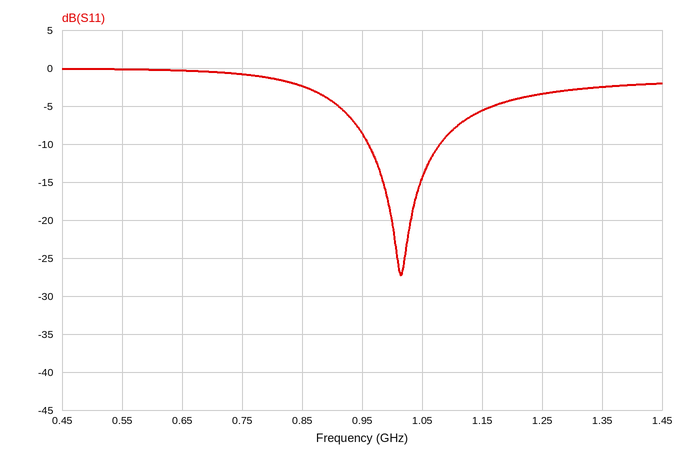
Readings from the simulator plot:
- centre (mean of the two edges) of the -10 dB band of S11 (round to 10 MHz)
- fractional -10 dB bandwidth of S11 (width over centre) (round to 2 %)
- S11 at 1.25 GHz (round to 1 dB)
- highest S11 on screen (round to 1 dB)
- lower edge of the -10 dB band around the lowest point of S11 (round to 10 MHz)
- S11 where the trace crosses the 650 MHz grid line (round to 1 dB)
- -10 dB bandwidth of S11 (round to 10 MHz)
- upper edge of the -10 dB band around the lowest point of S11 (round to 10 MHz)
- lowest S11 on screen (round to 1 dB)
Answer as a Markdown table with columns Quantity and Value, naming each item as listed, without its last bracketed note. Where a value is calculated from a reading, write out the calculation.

| Quantity | Value |
|---|---|
| centre (mean of the two edges) of the -10 dB band of S11 | 1.02 GHz |
| fractional -10 dB bandwidth of S11 (width over centre) | 120 MHz / 1.02 GHz ≈ 12 % |
| S11 at 1.25 GHz | -3 dB |
| highest S11 on screen | 0 dB |
| lower edge of the -10 dB band around the lowest point of S11 | 960 MHz |
| S11 where the trace crosses the 650 MHz grid line | 0 dB |
| -10 dB bandwidth of S11 | 1.08 GHz − 960 MHz = 120 MHz |
| upper edge of the -10 dB band around the lowest point of S11 | 1.08 GHz |
| lowest S11 on screen | -27 dB |
